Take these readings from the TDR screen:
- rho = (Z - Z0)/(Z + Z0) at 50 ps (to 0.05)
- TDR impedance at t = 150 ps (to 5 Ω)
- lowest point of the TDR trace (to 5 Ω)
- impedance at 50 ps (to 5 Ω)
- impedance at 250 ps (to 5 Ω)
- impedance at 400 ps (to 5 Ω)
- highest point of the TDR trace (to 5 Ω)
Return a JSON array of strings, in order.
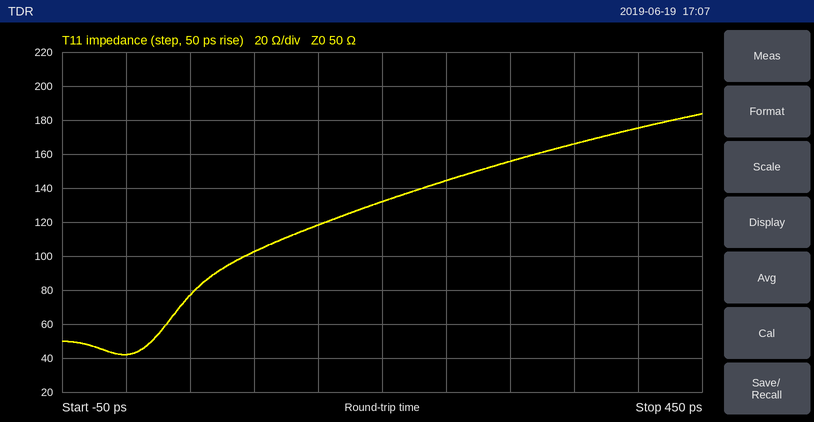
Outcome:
["+0.20", "120 Ω", "40 Ω", "75 Ω", "145 Ω", "175 Ω", "185 Ω"]
